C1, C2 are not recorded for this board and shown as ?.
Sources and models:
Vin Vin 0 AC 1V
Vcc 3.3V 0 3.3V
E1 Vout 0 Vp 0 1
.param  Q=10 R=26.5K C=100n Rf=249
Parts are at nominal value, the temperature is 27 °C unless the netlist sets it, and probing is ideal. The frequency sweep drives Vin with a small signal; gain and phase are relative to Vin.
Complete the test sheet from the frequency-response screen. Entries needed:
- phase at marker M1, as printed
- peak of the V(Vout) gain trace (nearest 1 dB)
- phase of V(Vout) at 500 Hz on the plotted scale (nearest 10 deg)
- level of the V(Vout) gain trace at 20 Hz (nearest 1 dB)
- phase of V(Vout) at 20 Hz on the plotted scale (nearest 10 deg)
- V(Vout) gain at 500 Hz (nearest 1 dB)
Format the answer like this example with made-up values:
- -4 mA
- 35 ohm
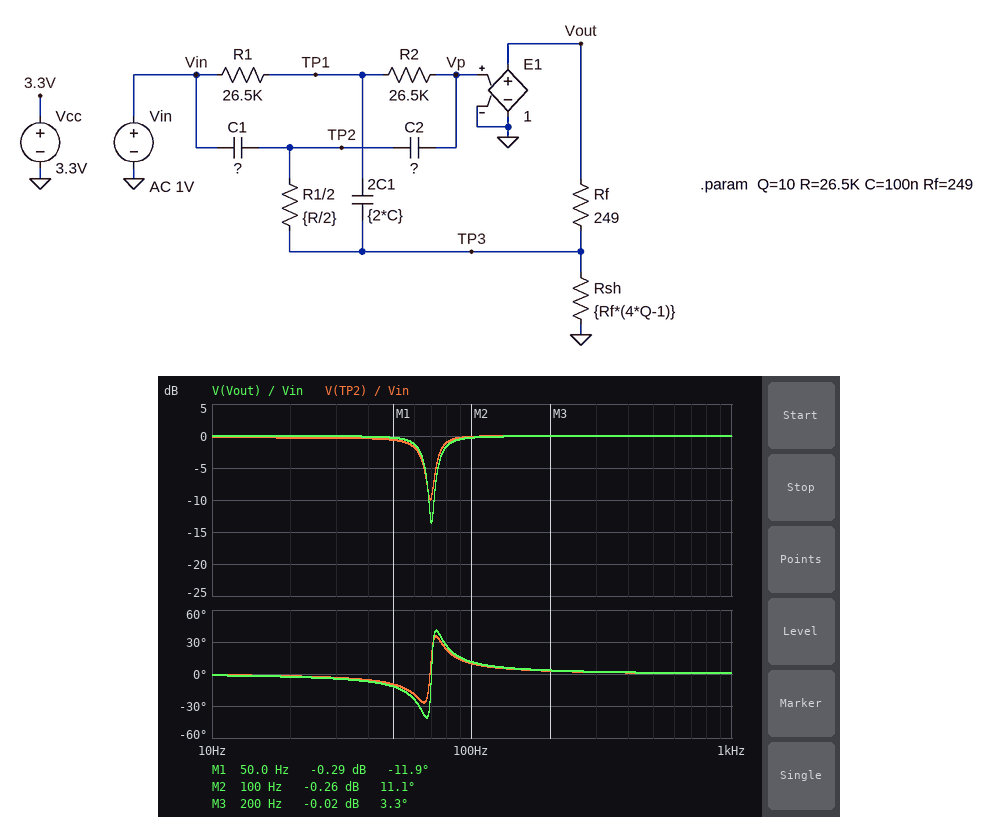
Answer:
- -11.9 deg
- 0 dB
- 0 deg
- 0 dB
- 0 deg
- 0 dB
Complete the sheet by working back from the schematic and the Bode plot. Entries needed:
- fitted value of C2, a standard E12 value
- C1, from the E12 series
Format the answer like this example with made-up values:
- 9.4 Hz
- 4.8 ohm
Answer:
- 150 nF
- 47 nF
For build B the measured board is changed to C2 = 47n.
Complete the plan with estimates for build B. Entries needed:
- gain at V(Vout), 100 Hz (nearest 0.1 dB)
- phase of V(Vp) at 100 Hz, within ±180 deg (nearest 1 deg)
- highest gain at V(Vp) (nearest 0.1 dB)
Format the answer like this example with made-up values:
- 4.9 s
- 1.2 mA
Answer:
- 5.4 dB
- -5 deg
- 5.5 dB
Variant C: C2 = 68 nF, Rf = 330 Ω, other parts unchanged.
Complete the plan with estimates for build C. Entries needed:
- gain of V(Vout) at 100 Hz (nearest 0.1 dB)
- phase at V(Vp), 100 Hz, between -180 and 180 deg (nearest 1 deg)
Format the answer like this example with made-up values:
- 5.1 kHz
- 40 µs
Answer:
- 1.9 dB
- 34 deg
